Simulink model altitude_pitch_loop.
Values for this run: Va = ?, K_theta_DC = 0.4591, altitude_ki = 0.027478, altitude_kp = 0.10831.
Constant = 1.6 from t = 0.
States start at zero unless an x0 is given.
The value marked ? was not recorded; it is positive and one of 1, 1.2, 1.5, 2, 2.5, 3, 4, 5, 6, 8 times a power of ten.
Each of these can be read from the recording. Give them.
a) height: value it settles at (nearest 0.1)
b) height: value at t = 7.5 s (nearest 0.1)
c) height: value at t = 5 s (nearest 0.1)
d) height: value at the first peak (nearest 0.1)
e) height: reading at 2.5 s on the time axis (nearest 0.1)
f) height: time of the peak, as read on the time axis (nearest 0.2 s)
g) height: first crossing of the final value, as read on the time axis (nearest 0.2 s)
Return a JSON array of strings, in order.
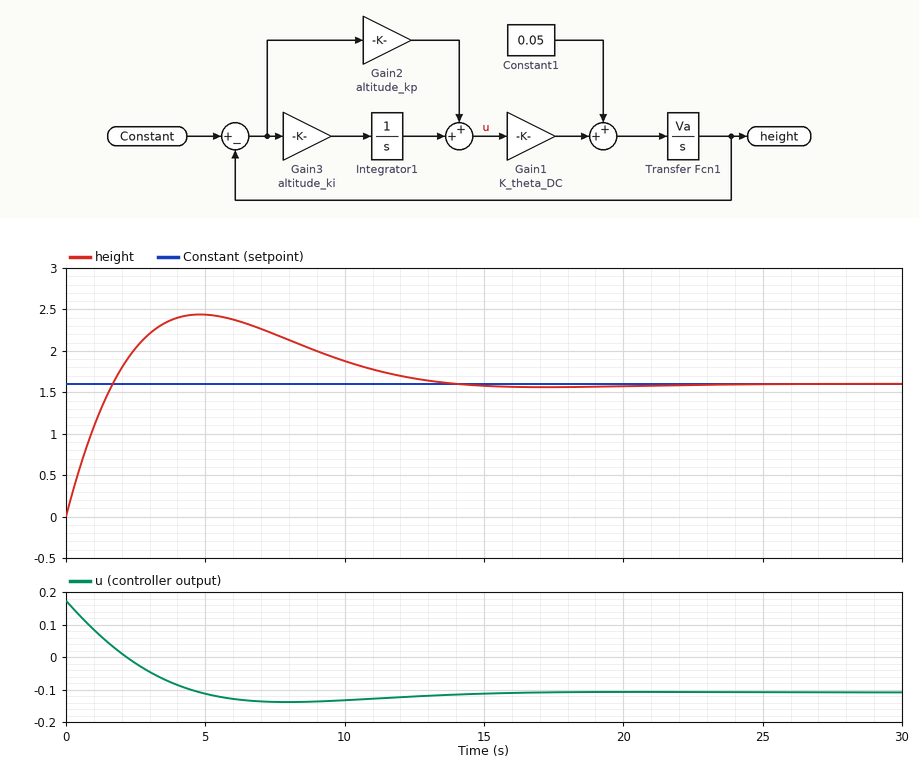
["1.6", "2.2", "2.4", "2.4", "2.0", "4.8 s", "1.6 s"]
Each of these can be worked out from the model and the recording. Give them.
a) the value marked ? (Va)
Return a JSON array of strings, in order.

["10"]
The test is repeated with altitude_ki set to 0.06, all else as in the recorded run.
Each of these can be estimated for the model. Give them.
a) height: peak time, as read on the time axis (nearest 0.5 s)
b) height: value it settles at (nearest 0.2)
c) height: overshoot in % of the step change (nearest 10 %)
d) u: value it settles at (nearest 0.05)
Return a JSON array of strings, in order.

["4.0 s", "1.6", "50 %", "-0.10"]
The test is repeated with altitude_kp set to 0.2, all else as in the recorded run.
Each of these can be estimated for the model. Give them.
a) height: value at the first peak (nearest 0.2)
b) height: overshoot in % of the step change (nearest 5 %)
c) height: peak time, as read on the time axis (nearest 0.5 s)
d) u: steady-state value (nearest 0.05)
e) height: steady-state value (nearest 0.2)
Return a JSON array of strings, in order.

["2.2", "35 %", "4.0 s", "-0.10", "1.6"]
